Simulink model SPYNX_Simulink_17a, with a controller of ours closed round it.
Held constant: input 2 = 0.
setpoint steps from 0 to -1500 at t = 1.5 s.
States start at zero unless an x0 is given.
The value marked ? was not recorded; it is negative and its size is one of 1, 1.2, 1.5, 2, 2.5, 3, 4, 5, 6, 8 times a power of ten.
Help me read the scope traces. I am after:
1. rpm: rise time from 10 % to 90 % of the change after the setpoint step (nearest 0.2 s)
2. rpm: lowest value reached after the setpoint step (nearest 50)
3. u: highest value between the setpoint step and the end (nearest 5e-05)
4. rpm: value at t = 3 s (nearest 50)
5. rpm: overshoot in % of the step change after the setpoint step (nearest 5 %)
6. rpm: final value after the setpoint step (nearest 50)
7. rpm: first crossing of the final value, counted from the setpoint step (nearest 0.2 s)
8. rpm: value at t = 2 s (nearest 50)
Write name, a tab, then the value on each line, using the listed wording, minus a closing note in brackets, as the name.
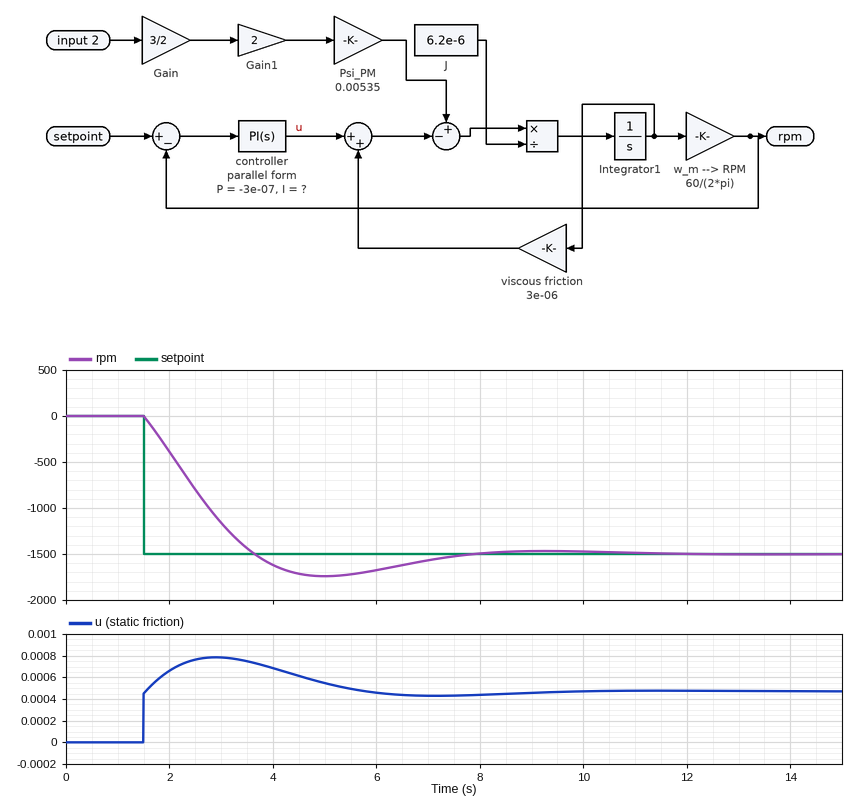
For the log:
rpm: rise time from 10 % to 90 % of the change after the setpoint step	1.6 s
rpm: lowest value reached after the setpoint step	-1750
u: highest value between the setpoint step and the end	0.00080
rpm: value at t = 3 s	-1150
rpm: overshoot in % of the step change after the setpoint step	15 %
rpm: final value after the setpoint step	-1500
rpm: first crossing of the final value, counted from the setpoint step	2.2 s
rpm: value at t = 2 s	-400
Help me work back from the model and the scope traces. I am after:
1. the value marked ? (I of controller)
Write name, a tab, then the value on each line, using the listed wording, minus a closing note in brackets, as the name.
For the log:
the value marked ?	-5e-07
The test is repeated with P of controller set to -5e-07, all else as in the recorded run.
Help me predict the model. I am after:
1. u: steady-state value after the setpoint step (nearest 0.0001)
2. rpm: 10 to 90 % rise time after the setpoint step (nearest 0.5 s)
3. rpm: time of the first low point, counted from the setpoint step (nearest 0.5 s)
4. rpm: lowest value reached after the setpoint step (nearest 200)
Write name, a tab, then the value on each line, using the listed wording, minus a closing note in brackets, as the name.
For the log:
u: steady-state value after the setpoint step	0.0005
rpm: 10 to 90 % rise time after the setpoint step	1.5 s
rpm: time of the first low point, counted from the setpoint step	3.5 s
rpm: lowest value reached after the setpoint step	-1600
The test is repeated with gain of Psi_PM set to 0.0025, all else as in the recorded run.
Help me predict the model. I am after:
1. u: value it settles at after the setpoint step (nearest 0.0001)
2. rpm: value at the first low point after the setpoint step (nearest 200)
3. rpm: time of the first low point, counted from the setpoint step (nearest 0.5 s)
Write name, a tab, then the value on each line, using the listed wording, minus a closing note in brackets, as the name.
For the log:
u: value it settles at after the setpoint step	0.0005
rpm: value at the first low point after the setpoint step	-1800
rpm: time of the first low point, counted from the setpoint step	3.5 s
